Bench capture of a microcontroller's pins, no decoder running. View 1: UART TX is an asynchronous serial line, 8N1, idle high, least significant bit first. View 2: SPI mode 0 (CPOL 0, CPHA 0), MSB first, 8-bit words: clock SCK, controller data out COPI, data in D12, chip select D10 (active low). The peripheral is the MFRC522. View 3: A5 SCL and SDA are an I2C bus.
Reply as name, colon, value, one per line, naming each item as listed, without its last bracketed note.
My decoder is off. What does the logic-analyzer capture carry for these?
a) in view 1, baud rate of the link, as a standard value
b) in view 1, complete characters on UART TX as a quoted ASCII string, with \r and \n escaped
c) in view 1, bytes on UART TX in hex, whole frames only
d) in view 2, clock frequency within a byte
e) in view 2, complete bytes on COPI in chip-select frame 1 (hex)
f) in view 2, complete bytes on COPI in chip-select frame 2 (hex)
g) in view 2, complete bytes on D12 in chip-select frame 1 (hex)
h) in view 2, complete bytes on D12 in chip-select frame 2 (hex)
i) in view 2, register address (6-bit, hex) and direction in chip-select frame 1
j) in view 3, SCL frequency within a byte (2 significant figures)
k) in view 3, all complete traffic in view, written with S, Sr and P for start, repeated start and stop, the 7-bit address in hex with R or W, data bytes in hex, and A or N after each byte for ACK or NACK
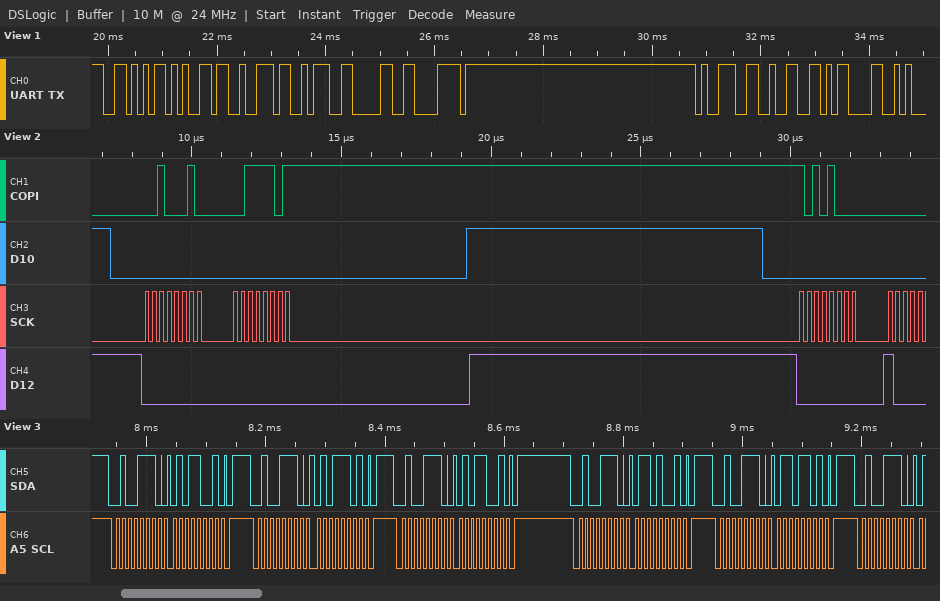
in view 1, baud rate of the link, as a standard value: 9600 baud
in view 1, complete characters on UART TX as a quoted ASCII string, with \r and \n escaped: "Ver:0x92\r"
in view 1, bytes on UART TX in hex, whole frames only: 0x56 0x65 0x72 0x3A 0x30 0x78 0x39 0x32 0x0D
in view 2, clock frequency within a byte: 4 MHz
in view 2, complete bytes on COPI in chip-select frame 1: 22 3D
in view 2, complete bytes on COPI in chip-select frame 2: A8
in view 2, complete bytes on D12 in chip-select frame 1: 00 00
in view 2, complete bytes on D12 in chip-select frame 2: 00
in view 2, register address (6-bit, hex) and direction in chip-select frame 1: 0x11 write
in view 3, SCL frequency within a byte: 100 kHz
in view 3, all complete traffic in view, written with S, Sr and P for start, repeated start and stop, the 7-bit address in hex with R or W, data bytes in hex, and A or N after each byte for ACK or NACK: S 27W A 59 A P S 27W A 5D A P S 27W A 59 A P S 27W A 69 A P S 27W A 6D A P S 27W A
